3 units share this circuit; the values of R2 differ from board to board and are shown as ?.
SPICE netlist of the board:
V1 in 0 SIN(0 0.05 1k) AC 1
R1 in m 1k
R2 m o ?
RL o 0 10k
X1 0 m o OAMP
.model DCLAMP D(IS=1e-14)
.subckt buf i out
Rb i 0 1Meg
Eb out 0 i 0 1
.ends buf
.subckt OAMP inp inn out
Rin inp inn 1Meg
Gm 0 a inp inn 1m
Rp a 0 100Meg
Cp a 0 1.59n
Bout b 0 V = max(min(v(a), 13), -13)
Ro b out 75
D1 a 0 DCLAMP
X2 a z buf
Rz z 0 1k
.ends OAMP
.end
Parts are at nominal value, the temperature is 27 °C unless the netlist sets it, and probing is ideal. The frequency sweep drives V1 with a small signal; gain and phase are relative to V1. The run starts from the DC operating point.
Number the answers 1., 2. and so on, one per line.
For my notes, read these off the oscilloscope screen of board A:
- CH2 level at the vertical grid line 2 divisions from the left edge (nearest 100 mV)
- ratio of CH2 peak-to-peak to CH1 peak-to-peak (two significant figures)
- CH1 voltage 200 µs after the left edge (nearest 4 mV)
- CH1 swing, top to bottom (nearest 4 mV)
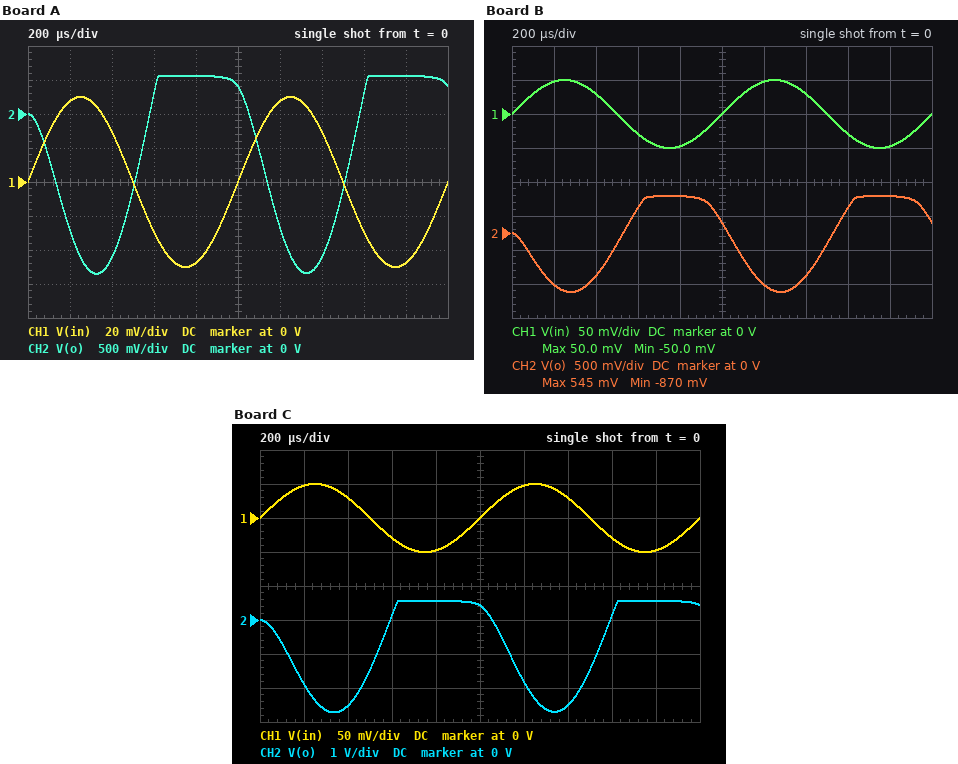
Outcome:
1. -2.1 V
2. 29
3. 48 mV
4. 100 mV
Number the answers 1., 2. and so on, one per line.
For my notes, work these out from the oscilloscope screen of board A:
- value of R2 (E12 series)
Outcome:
1. 56 kΩ
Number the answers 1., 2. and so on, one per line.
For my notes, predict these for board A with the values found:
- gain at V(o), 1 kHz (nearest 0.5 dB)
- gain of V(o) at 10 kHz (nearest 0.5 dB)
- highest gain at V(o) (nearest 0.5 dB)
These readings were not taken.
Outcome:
1. 33.5 dB
2. 19.5 dB
3. 34.5 dB
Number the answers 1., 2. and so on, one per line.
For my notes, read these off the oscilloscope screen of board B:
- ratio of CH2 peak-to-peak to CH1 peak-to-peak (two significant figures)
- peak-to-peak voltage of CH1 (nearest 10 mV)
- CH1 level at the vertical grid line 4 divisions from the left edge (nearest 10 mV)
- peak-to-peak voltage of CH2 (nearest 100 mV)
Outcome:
1. 14
2. 100 mV
3. -50 mV
4. 1.4 V
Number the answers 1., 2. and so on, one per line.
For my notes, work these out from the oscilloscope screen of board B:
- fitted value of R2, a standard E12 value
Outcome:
1. 18 kΩ
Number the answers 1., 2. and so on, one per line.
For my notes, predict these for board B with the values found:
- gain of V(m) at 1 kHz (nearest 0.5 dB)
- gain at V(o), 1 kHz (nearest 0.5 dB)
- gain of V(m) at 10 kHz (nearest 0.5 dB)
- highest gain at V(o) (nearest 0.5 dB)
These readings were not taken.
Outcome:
1. -15.0 dB
2. 25.0 dB
3. -1.5 dB
4. 25.0 dB
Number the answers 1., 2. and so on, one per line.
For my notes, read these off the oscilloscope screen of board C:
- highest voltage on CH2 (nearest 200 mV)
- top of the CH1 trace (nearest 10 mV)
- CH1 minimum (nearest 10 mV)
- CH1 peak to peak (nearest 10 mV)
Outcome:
1. 600 mV
2. 50 mV
3. -50 mV
4. 100 mV
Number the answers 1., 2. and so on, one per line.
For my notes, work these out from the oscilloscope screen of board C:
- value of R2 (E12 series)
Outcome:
1. 68 kΩ
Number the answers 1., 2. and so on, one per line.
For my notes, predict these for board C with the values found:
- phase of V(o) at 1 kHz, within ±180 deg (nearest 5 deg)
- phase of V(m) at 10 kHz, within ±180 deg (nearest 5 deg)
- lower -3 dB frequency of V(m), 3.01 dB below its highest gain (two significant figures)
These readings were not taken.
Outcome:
1. 145 deg
2. 10 deg
3. 1.5 kHz
